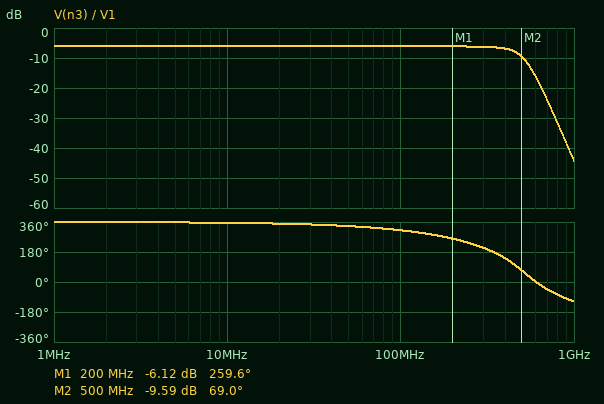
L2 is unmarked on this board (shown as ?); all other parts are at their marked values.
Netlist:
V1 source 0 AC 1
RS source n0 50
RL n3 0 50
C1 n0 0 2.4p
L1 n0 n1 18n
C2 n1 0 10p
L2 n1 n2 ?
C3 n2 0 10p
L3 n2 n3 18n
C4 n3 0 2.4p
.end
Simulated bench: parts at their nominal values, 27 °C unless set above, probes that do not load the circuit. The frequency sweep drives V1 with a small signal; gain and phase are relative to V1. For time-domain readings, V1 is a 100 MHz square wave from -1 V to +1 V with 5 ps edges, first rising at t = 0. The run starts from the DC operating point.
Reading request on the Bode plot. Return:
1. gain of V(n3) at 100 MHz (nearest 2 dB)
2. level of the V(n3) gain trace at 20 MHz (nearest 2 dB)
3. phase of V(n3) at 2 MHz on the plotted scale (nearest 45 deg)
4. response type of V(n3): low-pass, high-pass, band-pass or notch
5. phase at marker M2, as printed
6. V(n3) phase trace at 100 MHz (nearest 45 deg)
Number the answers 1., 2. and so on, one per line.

1. -6 dB
2. -6 dB
3. 360 deg
4. low-pass
5. 69.0 deg
6. 315 deg
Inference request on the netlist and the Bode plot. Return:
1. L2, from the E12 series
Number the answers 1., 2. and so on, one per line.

1. 39 nH
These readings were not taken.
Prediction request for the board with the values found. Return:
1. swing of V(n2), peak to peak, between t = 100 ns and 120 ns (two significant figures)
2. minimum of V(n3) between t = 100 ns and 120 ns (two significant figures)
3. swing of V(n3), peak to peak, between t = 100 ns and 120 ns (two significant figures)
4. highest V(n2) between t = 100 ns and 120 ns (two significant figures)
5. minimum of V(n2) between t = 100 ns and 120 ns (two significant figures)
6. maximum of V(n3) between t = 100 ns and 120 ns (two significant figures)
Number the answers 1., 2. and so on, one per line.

1. 1.3 V
2. -630 mV
3. 1.3 V
4. 670 mV
5. -670 mV
6. 630 mV
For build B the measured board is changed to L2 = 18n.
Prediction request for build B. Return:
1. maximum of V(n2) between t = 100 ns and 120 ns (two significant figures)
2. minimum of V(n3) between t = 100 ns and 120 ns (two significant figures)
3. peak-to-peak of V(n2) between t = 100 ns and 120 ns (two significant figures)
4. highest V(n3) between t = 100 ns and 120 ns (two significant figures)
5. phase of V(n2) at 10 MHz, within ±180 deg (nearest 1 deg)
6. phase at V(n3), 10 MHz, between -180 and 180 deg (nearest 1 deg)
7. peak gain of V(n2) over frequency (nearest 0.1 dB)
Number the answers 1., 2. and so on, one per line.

1. 730 mV
2. -650 mV
3. 1.5 V
4. 650 mV
5. -3 deg
6. -4 deg
7. -3.0 dB
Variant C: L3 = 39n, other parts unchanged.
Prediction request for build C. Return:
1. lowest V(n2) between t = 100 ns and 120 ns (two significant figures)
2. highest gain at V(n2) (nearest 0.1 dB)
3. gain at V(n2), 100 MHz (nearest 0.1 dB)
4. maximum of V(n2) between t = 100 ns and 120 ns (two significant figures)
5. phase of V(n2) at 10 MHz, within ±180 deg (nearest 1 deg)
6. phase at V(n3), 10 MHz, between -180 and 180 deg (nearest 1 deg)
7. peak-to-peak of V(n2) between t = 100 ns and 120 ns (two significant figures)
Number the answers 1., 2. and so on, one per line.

1. -910 mV
2. -0.5 dB
3. -5.5 dB
4. 910 mV
5. -3 deg
6. -6 deg
7. 1.8 V
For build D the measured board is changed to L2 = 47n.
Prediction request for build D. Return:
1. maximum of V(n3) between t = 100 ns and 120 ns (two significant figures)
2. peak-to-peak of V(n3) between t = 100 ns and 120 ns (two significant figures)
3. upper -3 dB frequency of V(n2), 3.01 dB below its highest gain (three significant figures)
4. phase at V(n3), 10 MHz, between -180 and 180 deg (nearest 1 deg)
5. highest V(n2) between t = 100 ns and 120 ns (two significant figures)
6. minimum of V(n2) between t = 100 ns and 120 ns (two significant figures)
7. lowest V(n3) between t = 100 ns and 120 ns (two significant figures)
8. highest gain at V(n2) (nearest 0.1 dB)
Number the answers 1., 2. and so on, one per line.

1. 600 mV
2. 1.2 V
3. 482 MHz
4. -5 deg
5. 630 mV
6. -630 mV
7. -600 mV
8. -6.0 dB
